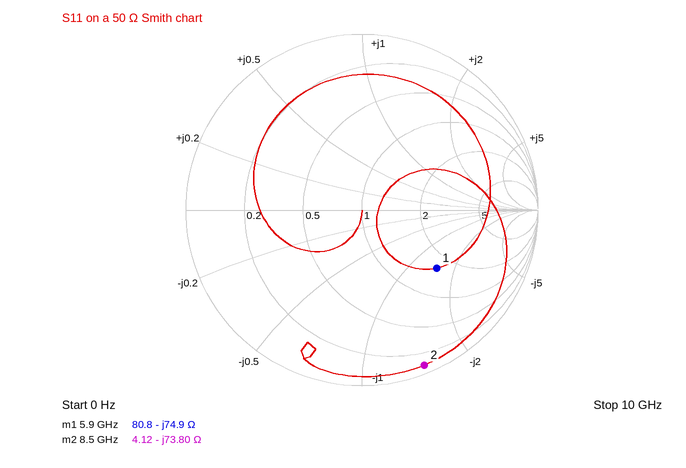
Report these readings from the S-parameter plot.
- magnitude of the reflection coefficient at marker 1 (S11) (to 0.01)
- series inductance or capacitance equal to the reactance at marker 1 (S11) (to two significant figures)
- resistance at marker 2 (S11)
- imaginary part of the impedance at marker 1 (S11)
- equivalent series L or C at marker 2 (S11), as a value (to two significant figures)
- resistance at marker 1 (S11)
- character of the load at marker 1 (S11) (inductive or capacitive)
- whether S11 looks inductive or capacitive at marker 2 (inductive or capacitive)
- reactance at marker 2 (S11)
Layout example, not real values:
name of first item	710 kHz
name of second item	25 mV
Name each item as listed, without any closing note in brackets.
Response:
magnitude of the reflection coefficient at marker 1 (S11)	0.54
series inductance or capacitance equal to the reactance at marker 1 (S11)	360 fF
resistance at marker 2	4.12 Ω
imaginary part of the impedance at marker 1	-74.9 Ω
equivalent series L or C at marker 2 (S11), as a value	250 fF
resistance at marker 1	80.8 Ω
character of the load at marker 1 (S11)	capacitive
whether S11 looks inductive or capacitive at marker 2	capacitive
reactance at marker 2	-73.80 Ω
